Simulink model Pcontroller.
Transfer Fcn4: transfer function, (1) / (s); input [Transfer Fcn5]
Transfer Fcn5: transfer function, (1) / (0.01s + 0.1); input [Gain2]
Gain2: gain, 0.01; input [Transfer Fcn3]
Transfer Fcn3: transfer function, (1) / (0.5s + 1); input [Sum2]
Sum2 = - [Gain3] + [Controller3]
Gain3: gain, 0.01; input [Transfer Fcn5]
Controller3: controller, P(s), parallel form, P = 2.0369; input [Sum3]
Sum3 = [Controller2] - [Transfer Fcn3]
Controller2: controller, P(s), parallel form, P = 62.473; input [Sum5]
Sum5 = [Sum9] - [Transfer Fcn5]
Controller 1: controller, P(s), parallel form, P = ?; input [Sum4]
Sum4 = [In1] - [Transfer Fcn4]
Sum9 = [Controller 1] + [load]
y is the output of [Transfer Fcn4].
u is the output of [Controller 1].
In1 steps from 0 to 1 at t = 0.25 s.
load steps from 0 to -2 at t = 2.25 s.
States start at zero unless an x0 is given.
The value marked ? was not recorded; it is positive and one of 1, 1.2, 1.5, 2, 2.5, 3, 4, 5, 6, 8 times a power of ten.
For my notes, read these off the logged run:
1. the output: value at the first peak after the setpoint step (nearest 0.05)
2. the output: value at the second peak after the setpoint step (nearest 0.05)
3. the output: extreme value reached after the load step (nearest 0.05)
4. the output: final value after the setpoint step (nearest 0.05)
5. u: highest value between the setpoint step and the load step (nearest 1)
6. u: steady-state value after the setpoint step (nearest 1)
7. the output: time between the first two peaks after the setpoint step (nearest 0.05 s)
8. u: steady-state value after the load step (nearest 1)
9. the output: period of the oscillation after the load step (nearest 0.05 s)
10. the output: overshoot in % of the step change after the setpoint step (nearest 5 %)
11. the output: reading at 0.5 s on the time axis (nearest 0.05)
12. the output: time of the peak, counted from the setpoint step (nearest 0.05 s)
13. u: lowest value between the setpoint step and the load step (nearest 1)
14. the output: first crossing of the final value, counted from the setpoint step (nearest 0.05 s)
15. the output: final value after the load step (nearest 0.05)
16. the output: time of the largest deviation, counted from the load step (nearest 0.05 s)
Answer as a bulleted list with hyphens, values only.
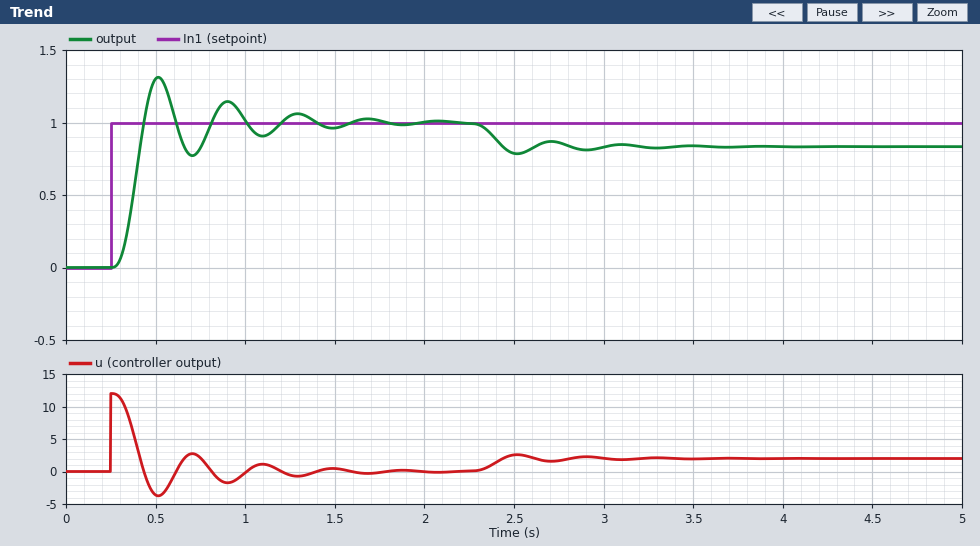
- 1.30
- 1.15
- 0.80
- 1.00
- 12
- 0
- 0.40 s
- 2
- 0.40 s
- 30 %
- 1.30
- 0.25 s
- -4
- 0.20 s
- 0.85
- 0.25 s
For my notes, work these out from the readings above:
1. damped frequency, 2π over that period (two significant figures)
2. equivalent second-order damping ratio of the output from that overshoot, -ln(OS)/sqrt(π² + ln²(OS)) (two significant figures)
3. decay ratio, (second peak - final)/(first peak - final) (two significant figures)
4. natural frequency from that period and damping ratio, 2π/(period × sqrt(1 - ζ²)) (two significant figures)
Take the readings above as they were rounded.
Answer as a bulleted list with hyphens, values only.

- 16 rad/s
- 0.36
- 0.50
- 17 rad/s
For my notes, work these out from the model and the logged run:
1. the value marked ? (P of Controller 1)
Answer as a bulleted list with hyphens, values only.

- 12
